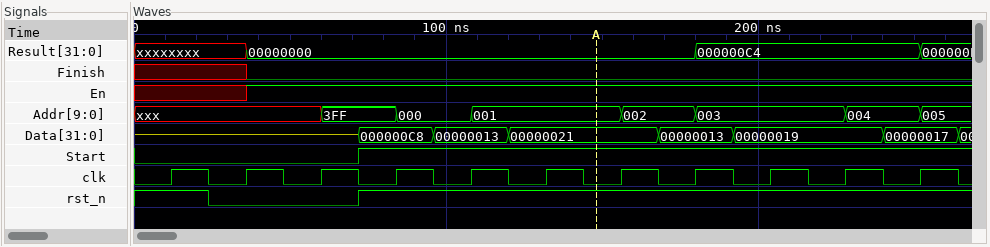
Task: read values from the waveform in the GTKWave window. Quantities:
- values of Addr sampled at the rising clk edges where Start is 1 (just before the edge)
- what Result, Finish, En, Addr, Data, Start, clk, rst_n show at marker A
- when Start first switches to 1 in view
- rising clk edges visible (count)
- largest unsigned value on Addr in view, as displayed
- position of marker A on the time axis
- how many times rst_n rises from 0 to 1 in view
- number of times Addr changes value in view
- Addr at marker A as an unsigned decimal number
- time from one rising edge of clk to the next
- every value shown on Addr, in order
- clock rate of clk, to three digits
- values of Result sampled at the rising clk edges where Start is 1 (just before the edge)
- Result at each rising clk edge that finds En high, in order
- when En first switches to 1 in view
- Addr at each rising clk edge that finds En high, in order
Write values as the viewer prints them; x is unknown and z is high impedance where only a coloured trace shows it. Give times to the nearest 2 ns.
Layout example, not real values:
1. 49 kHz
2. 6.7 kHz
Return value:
1. 3FF, 000, 001, 001, 002, 003, 003, 004
2. Result=00000000, Finish=0, En=1, Addr=001, Data=00000021, Start=1, clk=0, rst_n=1
3. 72 ns
4. 11
5. 3FF
6. 148 ns
7. 1
8. 7
9. 1
10. 24 ns
11. xxx, 3FF, 000, 001, 002, 003, 004, 005
12. 41.7 MHz
13. 00000000, 00000000, 00000000, 00000000, 00000000, 000000C4, 000000C4, 000000C4
14. 00000000, 00000000, 00000000, 00000000, 00000000, 00000000, 000000C4, 000000C4, 000000C4
15. 36 ns
16. xxx, 3FF, 000, 001, 001, 002, 003, 003, 004
